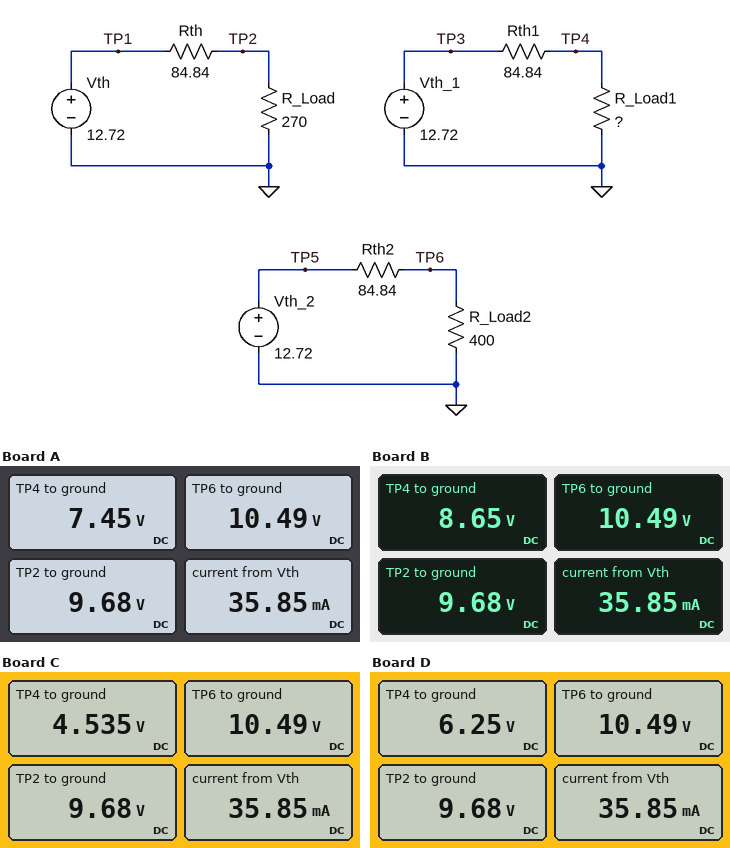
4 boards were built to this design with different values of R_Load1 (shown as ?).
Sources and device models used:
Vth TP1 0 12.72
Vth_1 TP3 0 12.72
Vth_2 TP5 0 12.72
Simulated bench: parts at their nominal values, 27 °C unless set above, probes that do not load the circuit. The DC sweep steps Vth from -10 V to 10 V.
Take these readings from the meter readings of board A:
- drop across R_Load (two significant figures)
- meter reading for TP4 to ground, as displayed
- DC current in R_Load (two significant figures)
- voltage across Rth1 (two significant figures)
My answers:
9.7 V
7.45 V
36 mA
5.3 V
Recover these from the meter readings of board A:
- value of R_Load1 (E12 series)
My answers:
120 Ω
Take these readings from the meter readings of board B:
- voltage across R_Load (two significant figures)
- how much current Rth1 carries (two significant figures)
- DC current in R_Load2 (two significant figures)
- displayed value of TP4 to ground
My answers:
9.7 V
48 mA
26 mA
8.65 V
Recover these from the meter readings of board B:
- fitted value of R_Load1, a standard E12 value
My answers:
180 Ω
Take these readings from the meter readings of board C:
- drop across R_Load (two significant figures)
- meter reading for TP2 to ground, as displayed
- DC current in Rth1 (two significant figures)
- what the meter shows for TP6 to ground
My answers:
9.7 V
9.68 V
96 mA
10.49 V
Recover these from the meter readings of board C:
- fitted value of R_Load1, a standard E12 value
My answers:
47 Ω
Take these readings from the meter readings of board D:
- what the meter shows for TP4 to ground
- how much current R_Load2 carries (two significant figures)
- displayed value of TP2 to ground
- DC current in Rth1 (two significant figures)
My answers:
6.25 V
26 mA
9.68 V
76 mA
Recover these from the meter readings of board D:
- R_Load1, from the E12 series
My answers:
82 Ω
